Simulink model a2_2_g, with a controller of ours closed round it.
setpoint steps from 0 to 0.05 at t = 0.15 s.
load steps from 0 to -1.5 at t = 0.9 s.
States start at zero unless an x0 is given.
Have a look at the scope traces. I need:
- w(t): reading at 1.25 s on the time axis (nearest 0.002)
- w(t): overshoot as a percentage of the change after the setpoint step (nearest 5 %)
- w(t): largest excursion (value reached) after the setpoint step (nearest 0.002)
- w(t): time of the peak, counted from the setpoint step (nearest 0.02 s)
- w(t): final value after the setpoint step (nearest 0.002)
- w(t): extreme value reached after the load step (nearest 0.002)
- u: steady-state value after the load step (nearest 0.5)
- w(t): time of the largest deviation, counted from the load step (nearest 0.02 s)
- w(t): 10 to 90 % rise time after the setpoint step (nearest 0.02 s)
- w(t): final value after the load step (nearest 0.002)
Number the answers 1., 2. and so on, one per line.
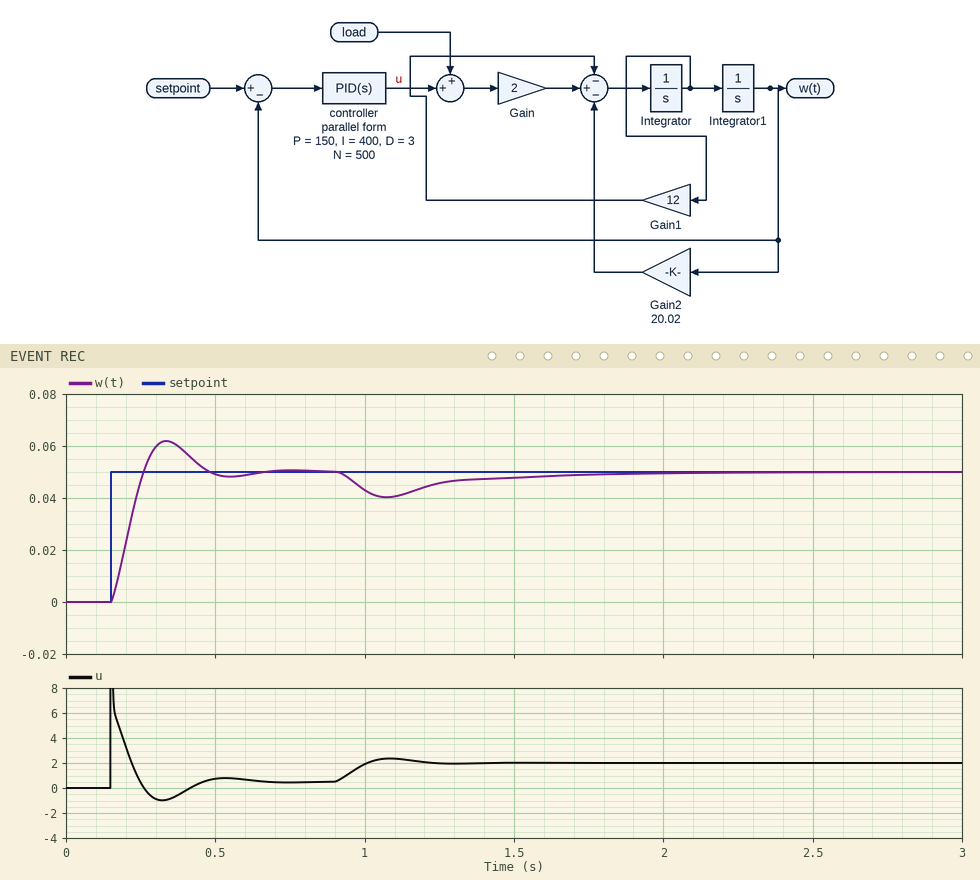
1. 0.046
2. 25 %
3. 0.062
4. 0.18 s
5. 0.050
6. 0.040
7. 2.0
8. 0.18 s
9. 0.08 s
10. 0.050
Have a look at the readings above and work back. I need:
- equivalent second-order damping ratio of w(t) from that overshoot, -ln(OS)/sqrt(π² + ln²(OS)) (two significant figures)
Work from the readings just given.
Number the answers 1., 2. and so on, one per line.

1. 0.40
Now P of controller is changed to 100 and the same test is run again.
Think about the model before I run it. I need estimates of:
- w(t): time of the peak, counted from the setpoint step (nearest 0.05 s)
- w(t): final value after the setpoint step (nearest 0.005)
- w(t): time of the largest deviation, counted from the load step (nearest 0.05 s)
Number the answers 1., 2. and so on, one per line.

1. 0.25 s
2. 0.050
3. 0.20 s
